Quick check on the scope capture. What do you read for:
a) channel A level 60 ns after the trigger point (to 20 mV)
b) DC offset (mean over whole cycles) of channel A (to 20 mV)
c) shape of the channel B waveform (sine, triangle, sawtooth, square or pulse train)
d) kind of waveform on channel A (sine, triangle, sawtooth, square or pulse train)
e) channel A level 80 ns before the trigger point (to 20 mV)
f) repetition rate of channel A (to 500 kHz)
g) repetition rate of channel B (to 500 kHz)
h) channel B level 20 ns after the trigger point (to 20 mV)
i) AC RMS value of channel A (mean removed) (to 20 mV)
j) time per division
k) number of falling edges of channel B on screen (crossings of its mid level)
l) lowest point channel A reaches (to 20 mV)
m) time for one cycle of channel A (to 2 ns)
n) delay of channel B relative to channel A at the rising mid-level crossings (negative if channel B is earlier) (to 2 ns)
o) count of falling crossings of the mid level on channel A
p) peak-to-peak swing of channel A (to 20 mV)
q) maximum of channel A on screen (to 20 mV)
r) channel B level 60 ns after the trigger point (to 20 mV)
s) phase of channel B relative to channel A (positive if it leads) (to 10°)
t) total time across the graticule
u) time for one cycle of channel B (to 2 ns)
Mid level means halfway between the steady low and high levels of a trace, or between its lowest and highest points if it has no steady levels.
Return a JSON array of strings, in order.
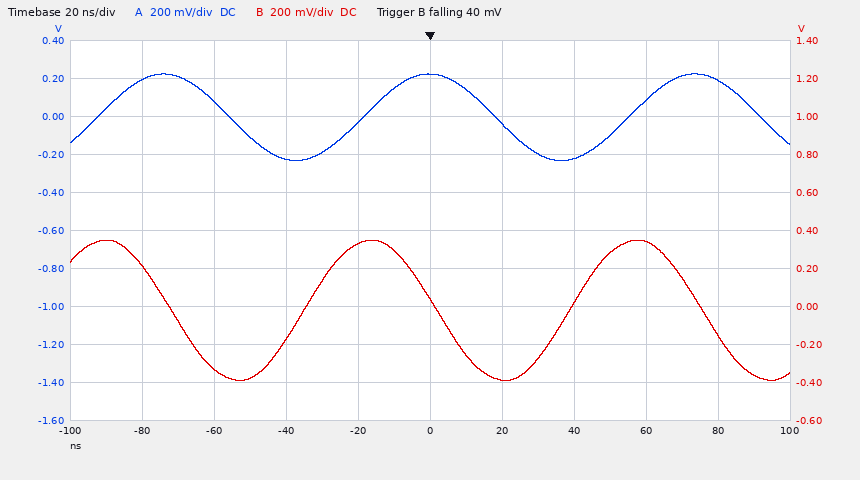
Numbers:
["80 mV", "0 mV", "sine", "sine", "200 mV", "13.5 MHz", "13.5 MHz", "-380 mV", "160 mV", "20 ns", "3", "-240 mV", "74 ns", "-16 ns", "3", "460 mV", "220 mV", "340 mV", "+80°", "200 ns", "74 ns"]
